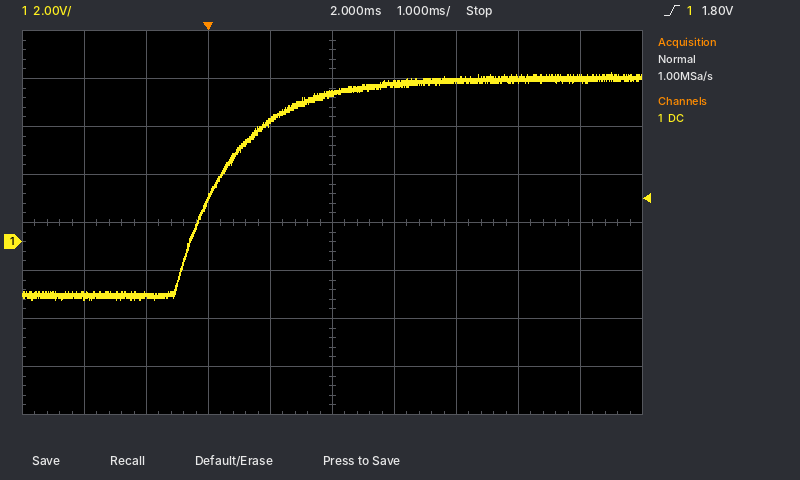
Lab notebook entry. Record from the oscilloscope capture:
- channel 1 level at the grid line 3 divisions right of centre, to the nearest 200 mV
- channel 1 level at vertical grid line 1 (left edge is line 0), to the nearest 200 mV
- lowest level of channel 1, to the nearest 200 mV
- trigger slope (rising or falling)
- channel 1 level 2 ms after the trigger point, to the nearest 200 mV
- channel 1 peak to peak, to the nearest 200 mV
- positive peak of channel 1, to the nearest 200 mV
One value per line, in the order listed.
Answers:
6.8 V
-2.2 V
-2.4 V
rising
6.2 V
9.4 V
7.0 V
